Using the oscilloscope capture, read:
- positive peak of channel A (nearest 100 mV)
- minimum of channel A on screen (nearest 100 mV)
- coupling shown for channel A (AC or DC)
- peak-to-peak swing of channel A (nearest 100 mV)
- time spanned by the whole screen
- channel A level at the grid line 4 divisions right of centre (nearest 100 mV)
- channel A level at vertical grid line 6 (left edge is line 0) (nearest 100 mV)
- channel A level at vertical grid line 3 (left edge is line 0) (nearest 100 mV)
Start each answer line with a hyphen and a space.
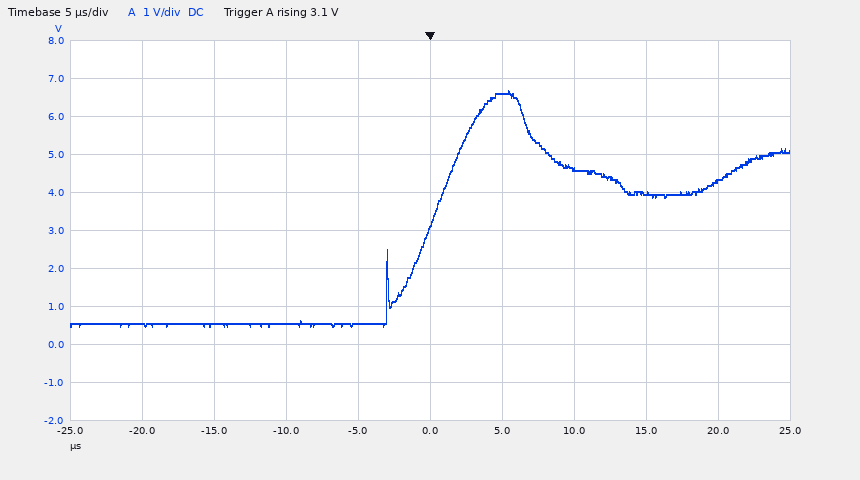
- 6.7 V
- 500 mV
- DC
- 6.2 V
- 50 µs
- 4.3 V
- 6.6 V
- 600 mV
